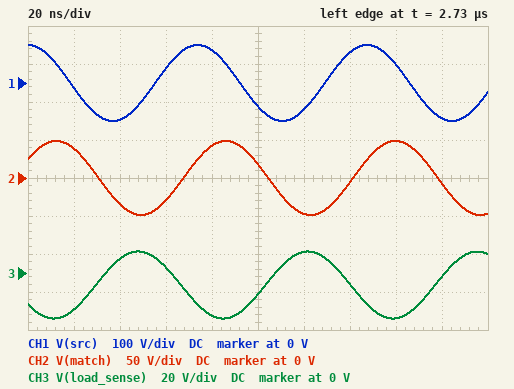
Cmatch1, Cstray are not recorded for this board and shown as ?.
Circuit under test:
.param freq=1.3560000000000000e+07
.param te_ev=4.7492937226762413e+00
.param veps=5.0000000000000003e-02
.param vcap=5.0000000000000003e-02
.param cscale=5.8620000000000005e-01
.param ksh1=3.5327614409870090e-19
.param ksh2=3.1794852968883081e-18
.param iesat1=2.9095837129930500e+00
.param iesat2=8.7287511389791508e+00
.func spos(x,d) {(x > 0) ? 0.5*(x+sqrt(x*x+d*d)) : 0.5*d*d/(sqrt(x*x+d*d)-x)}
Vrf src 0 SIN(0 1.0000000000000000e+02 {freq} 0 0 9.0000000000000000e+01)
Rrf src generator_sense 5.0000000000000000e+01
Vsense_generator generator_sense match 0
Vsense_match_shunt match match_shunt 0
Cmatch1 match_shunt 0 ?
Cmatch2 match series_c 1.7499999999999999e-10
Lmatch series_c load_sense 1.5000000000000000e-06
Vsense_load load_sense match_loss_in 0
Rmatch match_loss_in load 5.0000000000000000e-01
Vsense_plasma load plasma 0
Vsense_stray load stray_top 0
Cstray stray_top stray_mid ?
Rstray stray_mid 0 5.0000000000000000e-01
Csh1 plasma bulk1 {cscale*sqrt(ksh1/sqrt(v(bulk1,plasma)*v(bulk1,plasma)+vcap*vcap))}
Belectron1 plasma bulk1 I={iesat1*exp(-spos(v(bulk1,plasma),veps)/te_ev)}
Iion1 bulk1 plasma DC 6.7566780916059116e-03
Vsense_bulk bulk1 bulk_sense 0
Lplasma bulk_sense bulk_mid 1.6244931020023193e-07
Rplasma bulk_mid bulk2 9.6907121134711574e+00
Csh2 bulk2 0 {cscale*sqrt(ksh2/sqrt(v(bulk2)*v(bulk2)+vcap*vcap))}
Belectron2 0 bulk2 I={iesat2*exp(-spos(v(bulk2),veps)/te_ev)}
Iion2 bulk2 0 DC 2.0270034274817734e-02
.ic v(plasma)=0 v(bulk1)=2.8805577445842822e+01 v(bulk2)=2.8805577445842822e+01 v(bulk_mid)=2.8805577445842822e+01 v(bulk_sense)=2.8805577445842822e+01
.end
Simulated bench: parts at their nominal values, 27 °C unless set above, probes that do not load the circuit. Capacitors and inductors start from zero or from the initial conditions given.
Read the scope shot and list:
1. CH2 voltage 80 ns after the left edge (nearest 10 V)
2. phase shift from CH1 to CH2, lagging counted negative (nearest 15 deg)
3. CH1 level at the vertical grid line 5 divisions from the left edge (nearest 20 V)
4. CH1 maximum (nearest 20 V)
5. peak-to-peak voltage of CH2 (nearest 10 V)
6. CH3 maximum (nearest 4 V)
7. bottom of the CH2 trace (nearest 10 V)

40 V
-60 deg
-60 V
100 V
100 V
12 V
-50 V
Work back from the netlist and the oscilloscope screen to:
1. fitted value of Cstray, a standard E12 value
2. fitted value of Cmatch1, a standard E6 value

680 pF
680 pF
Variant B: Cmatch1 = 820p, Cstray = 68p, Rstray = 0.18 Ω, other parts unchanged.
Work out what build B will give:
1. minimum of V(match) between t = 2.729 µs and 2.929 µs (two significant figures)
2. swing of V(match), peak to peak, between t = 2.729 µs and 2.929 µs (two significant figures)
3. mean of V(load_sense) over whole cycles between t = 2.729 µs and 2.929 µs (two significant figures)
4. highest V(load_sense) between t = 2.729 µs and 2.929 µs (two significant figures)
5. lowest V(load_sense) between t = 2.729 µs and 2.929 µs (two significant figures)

-21 V
43 V
-25 V
22 V
-74 V
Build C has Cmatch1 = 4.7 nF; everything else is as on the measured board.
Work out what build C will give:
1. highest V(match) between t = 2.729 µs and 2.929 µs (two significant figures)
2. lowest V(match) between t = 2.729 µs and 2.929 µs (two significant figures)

5.3 V
-5.2 V
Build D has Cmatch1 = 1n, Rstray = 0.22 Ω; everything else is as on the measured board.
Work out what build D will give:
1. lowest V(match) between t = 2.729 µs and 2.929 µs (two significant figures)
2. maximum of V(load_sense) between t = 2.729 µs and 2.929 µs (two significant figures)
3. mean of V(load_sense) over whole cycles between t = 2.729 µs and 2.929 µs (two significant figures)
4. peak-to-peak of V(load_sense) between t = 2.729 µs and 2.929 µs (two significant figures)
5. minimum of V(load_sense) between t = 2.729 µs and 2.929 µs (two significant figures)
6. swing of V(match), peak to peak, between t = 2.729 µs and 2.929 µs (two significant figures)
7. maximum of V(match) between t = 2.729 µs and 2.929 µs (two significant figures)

-30 V
8.2 V
-2.9 V
22 V
-14 V
61 V
30 V
